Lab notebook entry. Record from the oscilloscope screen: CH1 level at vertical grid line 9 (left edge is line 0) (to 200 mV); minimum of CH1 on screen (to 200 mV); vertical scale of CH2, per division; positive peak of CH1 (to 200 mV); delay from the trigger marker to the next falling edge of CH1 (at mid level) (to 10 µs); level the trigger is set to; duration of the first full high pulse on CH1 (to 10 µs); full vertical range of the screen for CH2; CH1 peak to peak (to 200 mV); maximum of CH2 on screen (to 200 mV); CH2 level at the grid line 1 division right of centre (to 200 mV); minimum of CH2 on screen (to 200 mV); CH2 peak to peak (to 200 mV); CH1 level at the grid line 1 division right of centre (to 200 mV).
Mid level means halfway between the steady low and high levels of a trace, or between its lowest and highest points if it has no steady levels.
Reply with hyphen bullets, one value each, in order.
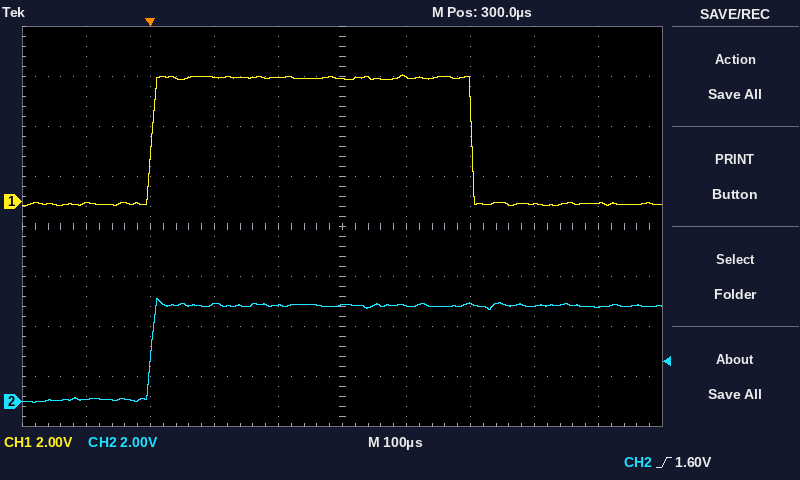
- 0.0 V
- -200 mV
- 2 V
- 5.0 V
- 500 µs
- 1.60 V
- 500 µs
- 16 V
- 5.2 V
- 4.2 V
- 3.8 V
- 0.0 V
- 4.2 V
- 5.0 V
